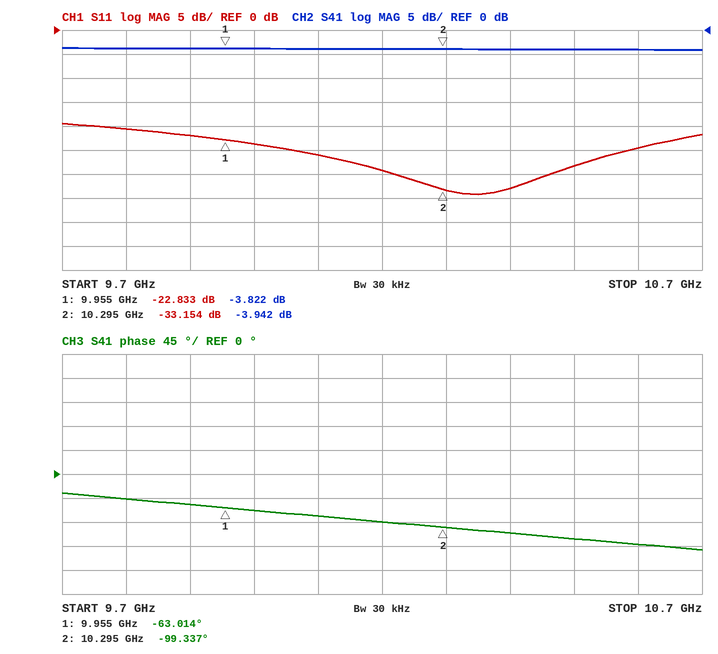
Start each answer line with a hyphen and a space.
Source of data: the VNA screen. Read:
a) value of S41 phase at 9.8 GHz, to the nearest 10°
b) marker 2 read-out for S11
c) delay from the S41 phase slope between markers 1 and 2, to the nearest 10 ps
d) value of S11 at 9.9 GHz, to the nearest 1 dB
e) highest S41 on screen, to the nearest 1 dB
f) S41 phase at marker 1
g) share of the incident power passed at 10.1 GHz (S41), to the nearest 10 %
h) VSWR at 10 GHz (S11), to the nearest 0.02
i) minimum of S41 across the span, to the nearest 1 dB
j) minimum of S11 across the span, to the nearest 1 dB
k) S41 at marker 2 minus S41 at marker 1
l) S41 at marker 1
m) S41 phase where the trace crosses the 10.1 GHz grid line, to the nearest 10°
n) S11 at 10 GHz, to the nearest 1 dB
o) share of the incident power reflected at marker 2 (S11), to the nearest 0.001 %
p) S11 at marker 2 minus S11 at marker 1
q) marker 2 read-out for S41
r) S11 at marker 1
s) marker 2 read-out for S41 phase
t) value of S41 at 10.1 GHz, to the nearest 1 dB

- -50°
- -33.154 dB
- 300 ps
- -22 dB
- -4 dB
- -63.014°
- 40 %
- 1.14
- -4 dB
- -34 dB
- -0.120 dB
- -3.822 dB
- -80°
- -24 dB
- 0.048 %
- -10.321 dB
- -3.942 dB
- -22.833 dB
- -99.337°
- -4 dB
